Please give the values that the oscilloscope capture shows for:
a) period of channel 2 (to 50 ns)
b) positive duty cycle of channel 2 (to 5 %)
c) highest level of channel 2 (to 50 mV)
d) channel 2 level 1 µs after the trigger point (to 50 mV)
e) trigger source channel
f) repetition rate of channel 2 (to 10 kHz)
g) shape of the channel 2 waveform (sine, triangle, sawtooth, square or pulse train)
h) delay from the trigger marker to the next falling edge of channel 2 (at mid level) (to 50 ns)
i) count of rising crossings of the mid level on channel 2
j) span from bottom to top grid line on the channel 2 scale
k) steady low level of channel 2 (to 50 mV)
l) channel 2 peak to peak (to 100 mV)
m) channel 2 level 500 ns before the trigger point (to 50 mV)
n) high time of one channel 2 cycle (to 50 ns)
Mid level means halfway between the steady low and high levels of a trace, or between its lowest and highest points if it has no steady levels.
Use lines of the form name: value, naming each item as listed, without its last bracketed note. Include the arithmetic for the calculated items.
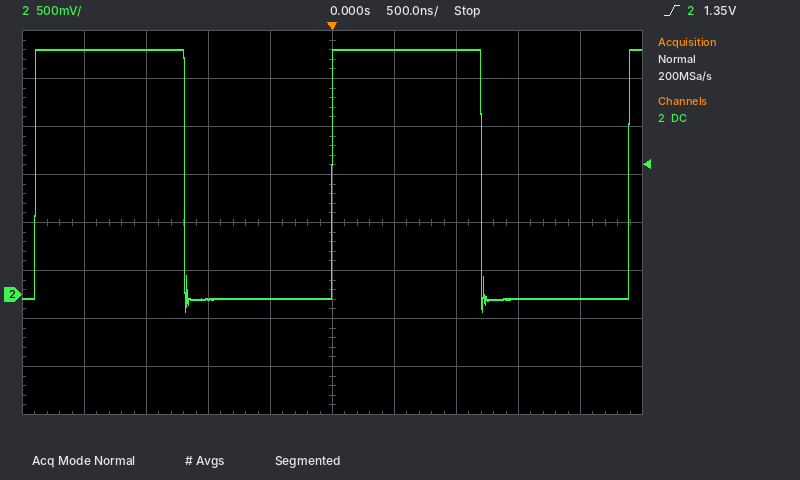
period of channel 2: 2.40 µs
positive duty cycle of channel 2: 1.20 µs / 2.40 µs ≈ 50 %
highest level of channel 2: 2.55 V
channel 2 level 1 µs after the trigger point: 2.55 V
trigger source channel: channel 2
repetition rate of channel 2: 1 / 2.40 µs ≈ 417 kHz, so 420 kHz to the nearest 10 kHz
shape of the channel 2 waveform: square
delay from the trigger marker to the next falling edge of channel 2 (at mid level): 1.20 µs
count of rising crossings of the mid level on channel 2: 3
span from bottom to top grid line on the channel 2 scale: 4 V
steady low level of channel 2: -50 mV
channel 2 peak to peak: 2.70 V
channel 2 level 500 ns before the trigger point: -50 mV
high time of one channel 2 cycle: 1.20 µs
